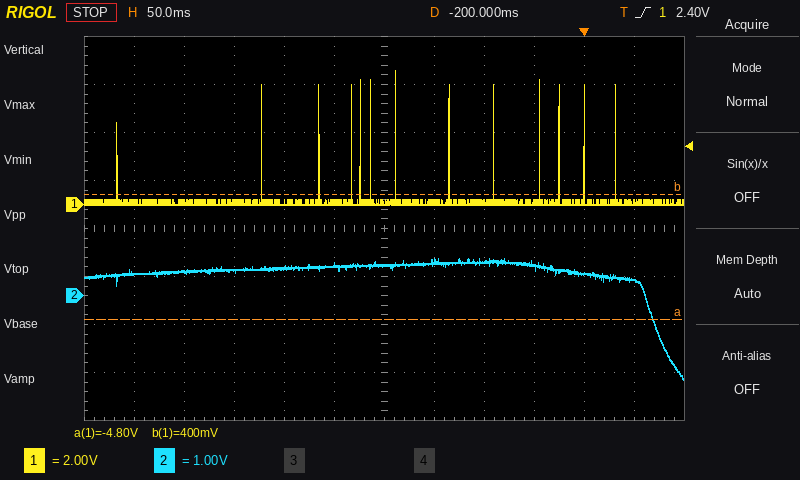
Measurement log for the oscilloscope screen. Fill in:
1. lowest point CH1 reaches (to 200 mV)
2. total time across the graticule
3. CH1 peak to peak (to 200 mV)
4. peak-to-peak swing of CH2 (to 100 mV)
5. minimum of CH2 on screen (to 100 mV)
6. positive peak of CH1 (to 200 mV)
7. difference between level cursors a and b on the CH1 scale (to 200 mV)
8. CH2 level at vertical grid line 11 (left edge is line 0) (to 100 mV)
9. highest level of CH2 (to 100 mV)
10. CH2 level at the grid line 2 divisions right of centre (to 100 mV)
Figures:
0.0 V
600 ms
5.6 V
2.5 V
-1.7 V
5.6 V
5.2 V
300 mV
800 mV
700 mV
